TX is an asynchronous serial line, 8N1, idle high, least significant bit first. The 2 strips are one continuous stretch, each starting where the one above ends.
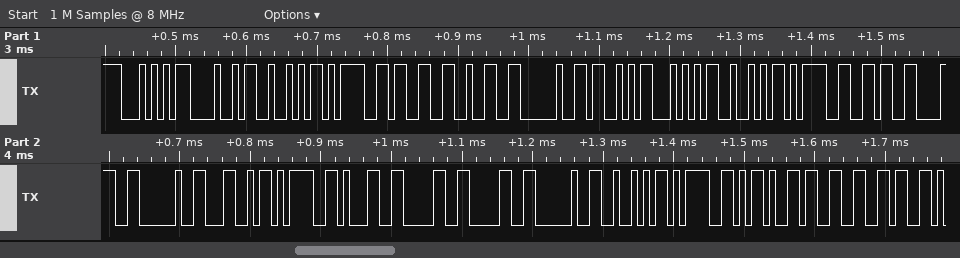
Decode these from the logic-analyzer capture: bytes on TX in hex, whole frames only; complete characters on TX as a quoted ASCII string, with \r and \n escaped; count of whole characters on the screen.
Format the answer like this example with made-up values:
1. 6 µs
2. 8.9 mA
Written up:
1. 54 48 52 3D 33 32 20 53 54 52 3D 36 38 20 4C 3D 31 30 30 20 52 3D 2D 33 36
2. "THR=32 STR=68 L=100 R=-36"
3. 25
